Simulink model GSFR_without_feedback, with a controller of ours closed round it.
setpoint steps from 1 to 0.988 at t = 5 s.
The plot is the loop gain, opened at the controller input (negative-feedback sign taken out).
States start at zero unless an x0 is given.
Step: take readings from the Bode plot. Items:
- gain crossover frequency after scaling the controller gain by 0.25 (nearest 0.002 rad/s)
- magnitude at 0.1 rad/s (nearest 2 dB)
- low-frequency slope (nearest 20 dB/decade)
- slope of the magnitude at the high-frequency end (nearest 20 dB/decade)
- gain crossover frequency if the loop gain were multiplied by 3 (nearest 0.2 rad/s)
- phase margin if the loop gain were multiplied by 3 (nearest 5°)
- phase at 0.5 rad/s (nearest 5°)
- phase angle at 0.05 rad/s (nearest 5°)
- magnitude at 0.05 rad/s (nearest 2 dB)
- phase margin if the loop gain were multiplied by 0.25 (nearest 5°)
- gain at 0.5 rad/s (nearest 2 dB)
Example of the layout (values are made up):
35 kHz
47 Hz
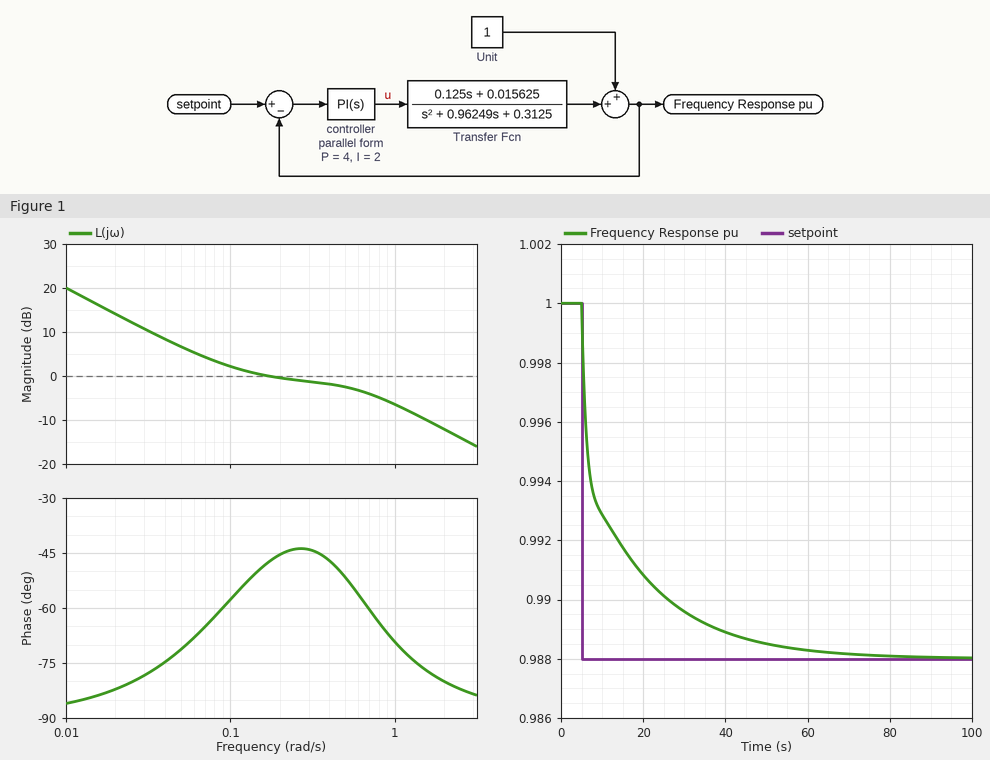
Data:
0.026 rad/s
2 dB
-20 dB/decade
-20 dB/decade
1.4 rad/s
105°
-50°
-70°
6 dB
100°
-2 dB
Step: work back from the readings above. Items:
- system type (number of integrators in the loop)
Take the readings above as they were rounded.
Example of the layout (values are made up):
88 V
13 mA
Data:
1
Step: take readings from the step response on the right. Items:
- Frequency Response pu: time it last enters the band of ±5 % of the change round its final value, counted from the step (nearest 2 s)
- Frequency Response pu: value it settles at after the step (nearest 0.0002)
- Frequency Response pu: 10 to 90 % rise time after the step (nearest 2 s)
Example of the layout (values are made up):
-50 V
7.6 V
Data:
42 s
0.9880
30 s
